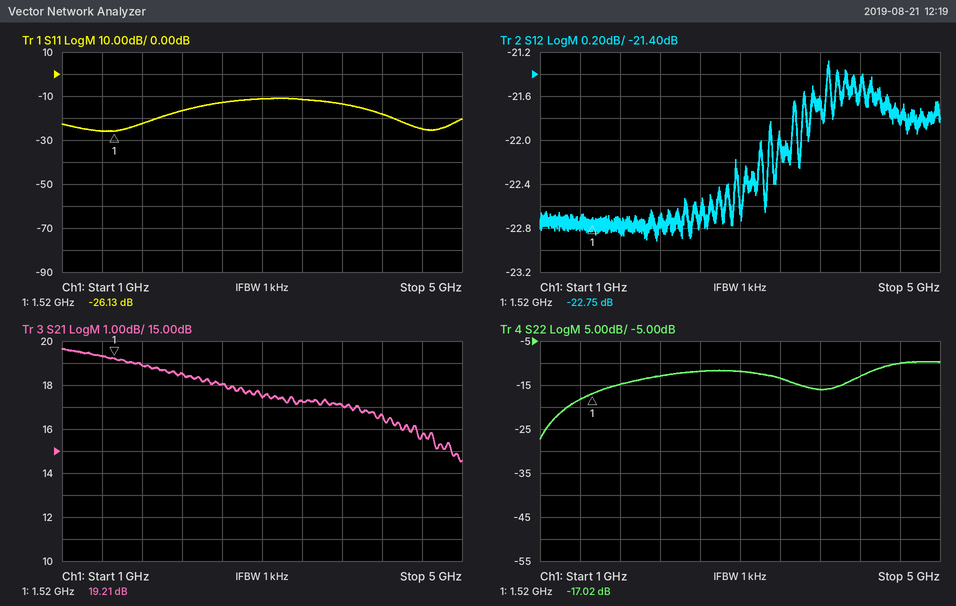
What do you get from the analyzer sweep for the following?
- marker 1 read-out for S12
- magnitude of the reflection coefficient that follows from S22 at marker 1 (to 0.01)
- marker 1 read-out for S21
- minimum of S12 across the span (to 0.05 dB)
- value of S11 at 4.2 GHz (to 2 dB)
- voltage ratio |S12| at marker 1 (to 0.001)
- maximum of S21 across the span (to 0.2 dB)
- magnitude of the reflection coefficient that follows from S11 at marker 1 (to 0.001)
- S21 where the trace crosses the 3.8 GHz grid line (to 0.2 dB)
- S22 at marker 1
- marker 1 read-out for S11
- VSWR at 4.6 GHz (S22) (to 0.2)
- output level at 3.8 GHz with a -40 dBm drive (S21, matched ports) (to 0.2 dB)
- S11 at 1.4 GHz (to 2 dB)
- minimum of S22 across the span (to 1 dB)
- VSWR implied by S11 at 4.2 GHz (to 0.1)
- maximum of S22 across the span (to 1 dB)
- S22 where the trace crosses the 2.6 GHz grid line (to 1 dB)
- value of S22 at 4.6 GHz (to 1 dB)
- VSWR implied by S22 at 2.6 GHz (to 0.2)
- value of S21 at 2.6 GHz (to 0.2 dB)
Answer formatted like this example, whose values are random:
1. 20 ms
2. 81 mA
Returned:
1. -22.75 dB
2. 0.14
3. 19.21 dB
4. -22.90 dB
5. -18 dB
6. 0.073
7. 19.6 dB
8. 0.049
9. 17.0 dB
10. -17.02 dB
11. -26.13 dB
12. 2.0
13. -23.0 dBm
14. -26 dB
15. -27 dB
16. 1.3
17. -10 dB
18. -12 dB
19. -10 dB
20. 1.6
21. 18.0 dB
